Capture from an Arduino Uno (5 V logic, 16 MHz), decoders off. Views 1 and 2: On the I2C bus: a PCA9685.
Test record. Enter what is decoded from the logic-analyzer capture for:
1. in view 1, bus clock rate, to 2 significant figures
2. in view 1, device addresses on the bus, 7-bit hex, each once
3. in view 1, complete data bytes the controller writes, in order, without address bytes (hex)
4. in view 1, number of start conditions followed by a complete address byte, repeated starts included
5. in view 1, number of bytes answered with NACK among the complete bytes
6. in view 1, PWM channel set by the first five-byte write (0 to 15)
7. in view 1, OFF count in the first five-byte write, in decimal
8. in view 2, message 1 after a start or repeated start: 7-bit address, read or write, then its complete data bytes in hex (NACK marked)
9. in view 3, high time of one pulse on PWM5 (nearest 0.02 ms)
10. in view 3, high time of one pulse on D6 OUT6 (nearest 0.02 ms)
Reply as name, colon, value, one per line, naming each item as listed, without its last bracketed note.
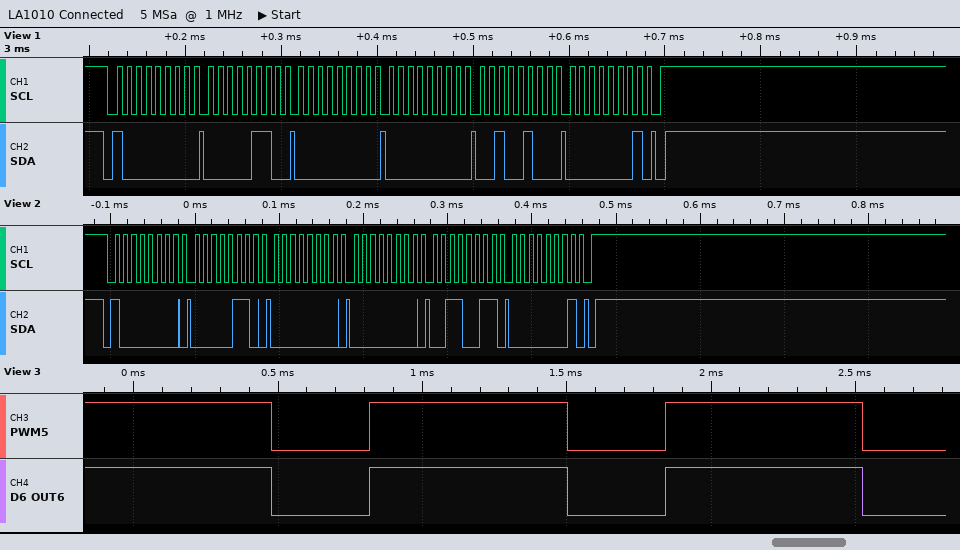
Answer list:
in view 1, bus clock rate, to 2 significant figures: 100 kHz
in view 1, device addresses on the bus, 7-bit hex, each once: 0x40
in view 1, complete data bytes the controller writes, in order, without address bytes: 06 00 00 24 01
in view 1, number of start conditions followed by a complete address byte, repeated starts included: 1
in view 1, number of bytes answered with NACK among the complete bytes: 0
in view 1, PWM channel set by the first five-byte write: 0
in view 1, OFF count in the first five-byte write, in decimal: 292
in view 2, message 1 after a start or repeated start: 7-bit address, read or write, then its complete data bytes in hex: 0x40 write: 06 00 00 33 01
in view 3, high time of one pulse on PWM5: 0.68 ms
in view 3, high time of one pulse on D6 OUT6: 0.68 ms
